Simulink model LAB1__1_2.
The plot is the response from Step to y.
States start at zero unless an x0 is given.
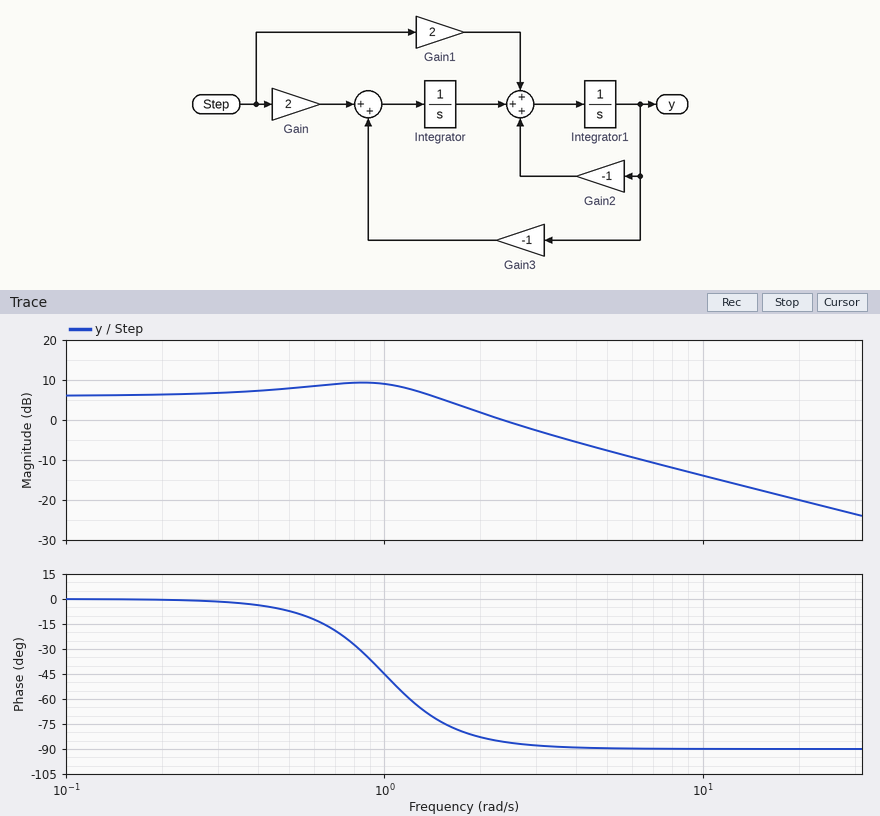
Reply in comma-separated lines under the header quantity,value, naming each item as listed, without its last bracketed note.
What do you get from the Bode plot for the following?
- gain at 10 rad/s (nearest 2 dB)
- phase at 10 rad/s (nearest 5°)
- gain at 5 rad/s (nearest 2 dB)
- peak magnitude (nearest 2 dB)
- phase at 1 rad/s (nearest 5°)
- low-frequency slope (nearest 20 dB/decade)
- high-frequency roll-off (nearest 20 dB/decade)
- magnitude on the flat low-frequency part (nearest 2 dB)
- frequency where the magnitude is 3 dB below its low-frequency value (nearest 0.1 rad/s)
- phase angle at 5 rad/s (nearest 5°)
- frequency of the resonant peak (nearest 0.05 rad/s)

quantity,value
gain at 10 rad/s,-14 dB
phase at 10 rad/s,-90°
gain at 5 rad/s,-8 dB
peak magnitude,10 dB
phase at 1 rad/s,-45°
low-frequency slope,0 dB/decade
high-frequency roll-off,-20 dB/decade
magnitude on the flat low-frequency part,6 dB
frequency where the magnitude is 3 dB below its low-frequency value,1.8 rad/s
phase angle at 5 rad/s,-90°
frequency of the resonant peak,0.85 rad/s
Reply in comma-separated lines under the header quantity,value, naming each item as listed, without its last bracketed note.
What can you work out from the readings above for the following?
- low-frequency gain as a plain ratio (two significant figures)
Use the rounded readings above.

quantity,value
low-frequency gain as a plain ratio,2.0
